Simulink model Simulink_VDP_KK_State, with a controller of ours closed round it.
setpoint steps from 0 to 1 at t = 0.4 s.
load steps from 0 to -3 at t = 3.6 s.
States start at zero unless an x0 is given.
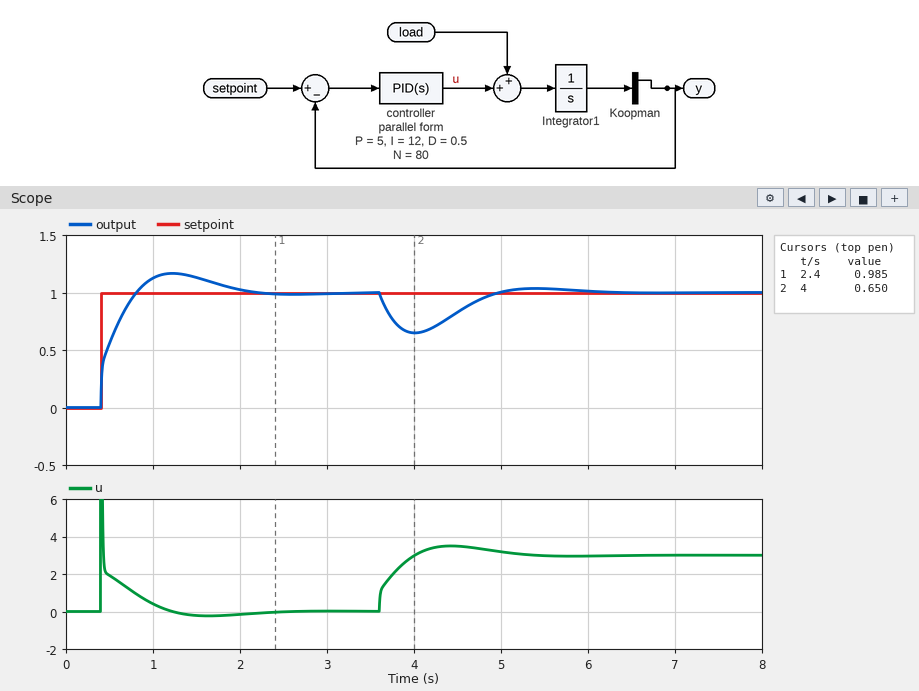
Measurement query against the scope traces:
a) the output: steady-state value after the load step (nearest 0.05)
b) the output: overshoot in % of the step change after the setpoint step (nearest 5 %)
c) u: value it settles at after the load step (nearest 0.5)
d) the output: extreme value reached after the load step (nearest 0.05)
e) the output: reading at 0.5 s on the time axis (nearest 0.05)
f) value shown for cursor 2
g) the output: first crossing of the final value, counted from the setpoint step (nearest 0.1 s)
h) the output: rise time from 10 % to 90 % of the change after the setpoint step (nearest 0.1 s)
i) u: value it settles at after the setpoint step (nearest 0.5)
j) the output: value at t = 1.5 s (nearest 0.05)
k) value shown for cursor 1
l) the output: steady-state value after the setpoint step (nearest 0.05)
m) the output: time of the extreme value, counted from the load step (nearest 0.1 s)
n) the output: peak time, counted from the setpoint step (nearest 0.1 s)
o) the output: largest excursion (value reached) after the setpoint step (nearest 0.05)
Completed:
1.00
15 %
3.0
0.65
0.55
0.650
0.4 s
0.3 s
0.0
1.15
0.985
1.00
0.4 s
0.8 s
1.15
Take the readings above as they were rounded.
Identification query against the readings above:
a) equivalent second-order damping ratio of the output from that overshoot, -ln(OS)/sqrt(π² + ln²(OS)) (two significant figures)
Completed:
0.52
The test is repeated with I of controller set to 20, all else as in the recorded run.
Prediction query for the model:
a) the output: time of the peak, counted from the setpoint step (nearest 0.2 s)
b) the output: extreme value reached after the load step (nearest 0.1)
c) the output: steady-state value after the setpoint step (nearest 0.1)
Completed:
0.6 s
0.7
1.0
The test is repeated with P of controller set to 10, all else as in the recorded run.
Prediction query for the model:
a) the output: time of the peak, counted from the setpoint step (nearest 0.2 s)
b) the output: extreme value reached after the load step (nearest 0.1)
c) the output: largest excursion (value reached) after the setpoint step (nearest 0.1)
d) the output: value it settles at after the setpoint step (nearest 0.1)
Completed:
0.6 s
0.8
1.1
1.0
